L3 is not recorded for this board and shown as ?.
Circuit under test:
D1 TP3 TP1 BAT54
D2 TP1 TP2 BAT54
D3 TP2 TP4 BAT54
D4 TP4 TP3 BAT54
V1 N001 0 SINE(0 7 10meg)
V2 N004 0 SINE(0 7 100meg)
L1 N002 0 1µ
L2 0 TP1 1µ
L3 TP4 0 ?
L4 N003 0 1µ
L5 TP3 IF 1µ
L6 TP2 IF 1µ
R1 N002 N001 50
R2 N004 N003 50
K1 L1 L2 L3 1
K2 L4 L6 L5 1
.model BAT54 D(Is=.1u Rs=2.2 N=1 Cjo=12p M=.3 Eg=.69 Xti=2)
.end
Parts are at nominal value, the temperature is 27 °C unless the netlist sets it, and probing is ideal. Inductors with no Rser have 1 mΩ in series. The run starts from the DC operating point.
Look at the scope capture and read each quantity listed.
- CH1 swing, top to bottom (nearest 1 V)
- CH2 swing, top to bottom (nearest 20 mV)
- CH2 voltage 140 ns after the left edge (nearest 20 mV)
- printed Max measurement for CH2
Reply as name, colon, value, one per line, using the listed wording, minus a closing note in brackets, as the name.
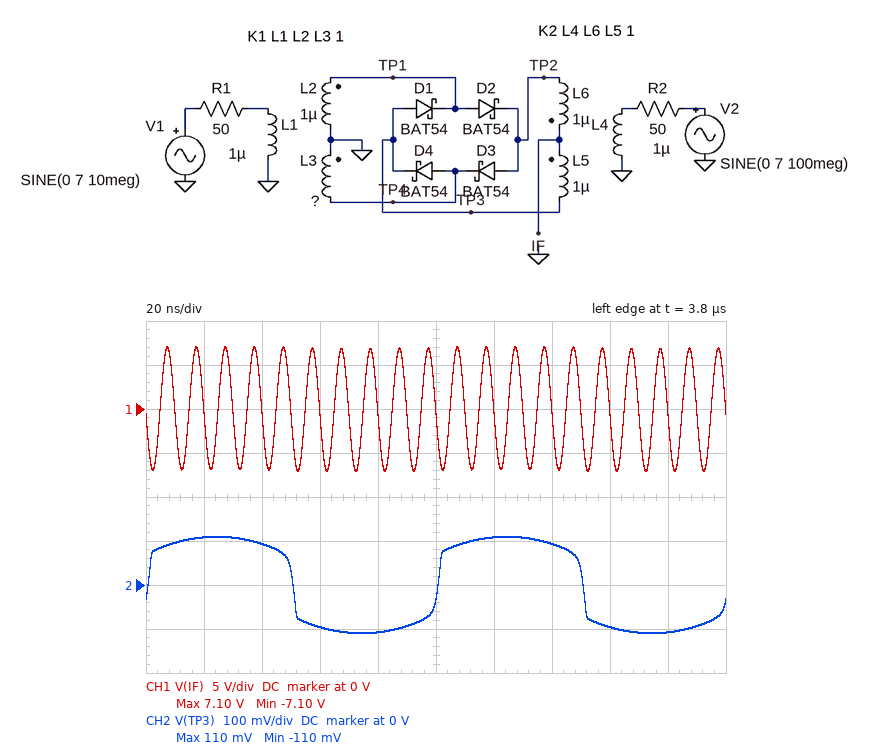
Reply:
CH1 swing, top to bottom: 14 V
CH2 swing, top to bottom: 220 mV
CH2 voltage 140 ns after the left edge: 100 mV
printed Max measurement for CH2: 110 mV
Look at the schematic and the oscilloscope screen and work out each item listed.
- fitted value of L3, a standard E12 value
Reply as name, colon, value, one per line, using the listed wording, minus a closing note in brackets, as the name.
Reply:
fitted value of L3, a standard E12 value: 2.7 µH
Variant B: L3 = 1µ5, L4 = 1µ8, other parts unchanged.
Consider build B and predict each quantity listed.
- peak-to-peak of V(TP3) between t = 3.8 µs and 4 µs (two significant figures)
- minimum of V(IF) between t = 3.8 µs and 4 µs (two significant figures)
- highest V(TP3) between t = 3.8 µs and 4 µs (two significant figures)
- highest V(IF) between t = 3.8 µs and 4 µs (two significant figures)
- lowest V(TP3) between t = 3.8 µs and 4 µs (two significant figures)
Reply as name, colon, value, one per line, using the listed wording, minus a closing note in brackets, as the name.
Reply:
peak-to-peak of V(TP3) between t = 3.8 µs and 4 µs: 96 mV
minimum of V(IF) between t = 3.8 µs and 4 µs: -5.3 V
highest V(TP3) between t = 3.8 µs and 4 µs: 48 mV
highest V(IF) between t = 3.8 µs and 4 µs: 5.3 V
lowest V(TP3) between t = 3.8 µs and 4 µs: -48 mV
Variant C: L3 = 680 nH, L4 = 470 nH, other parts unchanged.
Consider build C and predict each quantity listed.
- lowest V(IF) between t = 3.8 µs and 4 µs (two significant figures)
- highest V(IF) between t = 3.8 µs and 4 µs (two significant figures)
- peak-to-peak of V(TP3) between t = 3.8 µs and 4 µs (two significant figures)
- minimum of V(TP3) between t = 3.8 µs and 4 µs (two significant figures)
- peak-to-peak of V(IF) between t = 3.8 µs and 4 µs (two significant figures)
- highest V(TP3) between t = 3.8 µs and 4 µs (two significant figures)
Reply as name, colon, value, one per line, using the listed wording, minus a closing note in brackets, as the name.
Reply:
lowest V(IF) between t = 3.8 µs and 4 µs: -10 V
highest V(IF) between t = 3.8 µs and 4 µs: 10 V
peak-to-peak of V(TP3) between t = 3.8 µs and 4 µs: 97 mV
minimum of V(TP3) between t = 3.8 µs and 4 µs: -48 mV
peak-to-peak of V(IF) between t = 3.8 µs and 4 µs: 20 V
highest V(TP3) between t = 3.8 µs and 4 µs: 48 mV
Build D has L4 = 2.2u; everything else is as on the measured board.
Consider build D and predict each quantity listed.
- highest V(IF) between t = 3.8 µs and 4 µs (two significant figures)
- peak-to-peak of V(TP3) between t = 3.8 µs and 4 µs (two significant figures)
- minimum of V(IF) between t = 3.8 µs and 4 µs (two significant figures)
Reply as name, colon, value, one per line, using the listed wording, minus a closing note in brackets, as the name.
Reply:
highest V(IF) between t = 3.8 µs and 4 µs: 4.8 V
peak-to-peak of V(TP3) between t = 3.8 µs and 4 µs: 220 mV
minimum of V(IF) between t = 3.8 µs and 4 µs: -4.8 V
